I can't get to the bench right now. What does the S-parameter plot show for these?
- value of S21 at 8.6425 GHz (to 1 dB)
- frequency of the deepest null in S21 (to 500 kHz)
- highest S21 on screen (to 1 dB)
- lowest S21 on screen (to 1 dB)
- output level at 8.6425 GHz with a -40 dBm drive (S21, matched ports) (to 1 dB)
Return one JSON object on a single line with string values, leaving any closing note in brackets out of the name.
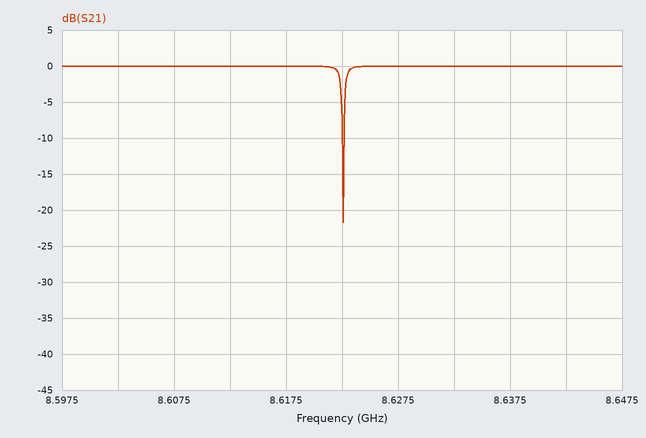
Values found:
{"value of S21 at 8.6425 GHz": "0 dB", "frequency of the deepest null in S21": "8.6225 GHz", "highest S21 on screen": "0 dB", "lowest S21 on screen": "-22 dB", "output level at 8.6425 GHz with a -40 dBm drive (S21, matched ports)": "-40 dBm"}
